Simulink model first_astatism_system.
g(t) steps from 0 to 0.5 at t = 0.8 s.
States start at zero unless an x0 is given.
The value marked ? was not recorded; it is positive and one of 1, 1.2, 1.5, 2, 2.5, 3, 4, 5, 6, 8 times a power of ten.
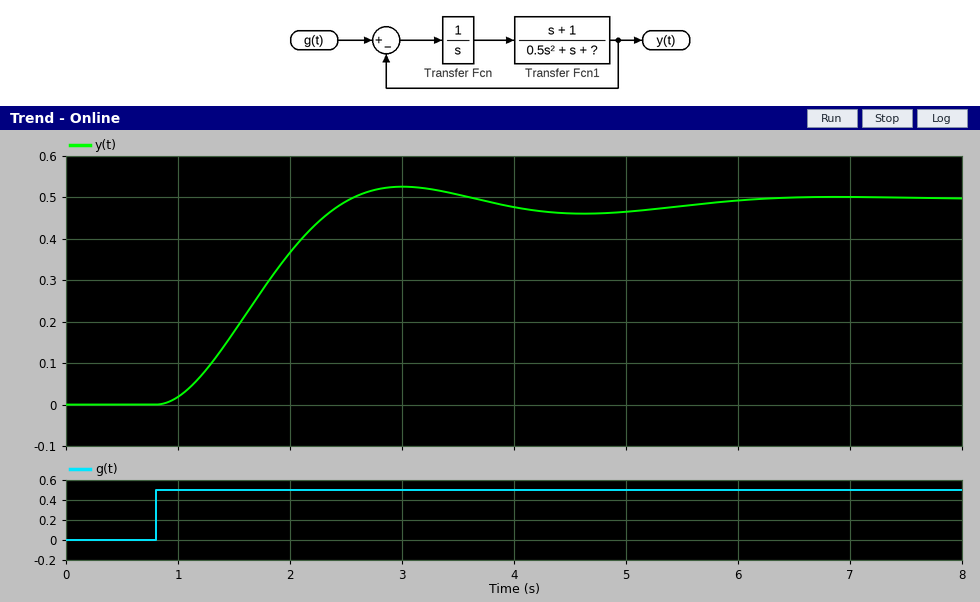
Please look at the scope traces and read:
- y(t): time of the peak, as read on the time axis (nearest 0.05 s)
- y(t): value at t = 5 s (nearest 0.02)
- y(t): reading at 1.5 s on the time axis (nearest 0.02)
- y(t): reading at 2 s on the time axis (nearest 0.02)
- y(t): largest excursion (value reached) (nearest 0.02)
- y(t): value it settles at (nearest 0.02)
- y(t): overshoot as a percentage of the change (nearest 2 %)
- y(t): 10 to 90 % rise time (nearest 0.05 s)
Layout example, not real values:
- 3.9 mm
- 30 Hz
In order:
- 3.00 s
- 0.46
- 0.18
- 0.36
- 0.52
- 0.50
- 6 %
- 1.15 s
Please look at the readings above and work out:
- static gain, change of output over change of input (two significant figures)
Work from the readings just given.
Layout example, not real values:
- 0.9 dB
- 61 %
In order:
- 1.0
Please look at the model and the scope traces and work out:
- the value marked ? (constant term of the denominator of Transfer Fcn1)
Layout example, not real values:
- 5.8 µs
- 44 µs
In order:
- 1
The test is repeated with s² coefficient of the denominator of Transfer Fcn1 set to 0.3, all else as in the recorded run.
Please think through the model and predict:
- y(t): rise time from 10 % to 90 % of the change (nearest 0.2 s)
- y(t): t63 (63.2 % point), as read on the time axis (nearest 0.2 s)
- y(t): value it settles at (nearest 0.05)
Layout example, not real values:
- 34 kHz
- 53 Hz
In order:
- 1.4 s
- 1.8 s
- 0.50
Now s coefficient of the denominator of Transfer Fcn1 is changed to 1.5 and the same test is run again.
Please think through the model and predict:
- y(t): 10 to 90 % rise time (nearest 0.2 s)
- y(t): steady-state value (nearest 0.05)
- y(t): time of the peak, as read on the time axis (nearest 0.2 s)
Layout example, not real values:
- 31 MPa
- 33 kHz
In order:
- 1.6 s
- 0.50
- 4.0 s
